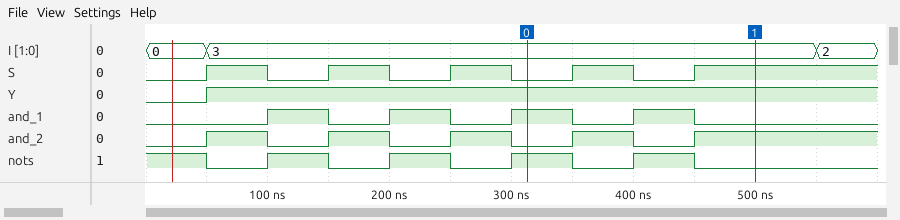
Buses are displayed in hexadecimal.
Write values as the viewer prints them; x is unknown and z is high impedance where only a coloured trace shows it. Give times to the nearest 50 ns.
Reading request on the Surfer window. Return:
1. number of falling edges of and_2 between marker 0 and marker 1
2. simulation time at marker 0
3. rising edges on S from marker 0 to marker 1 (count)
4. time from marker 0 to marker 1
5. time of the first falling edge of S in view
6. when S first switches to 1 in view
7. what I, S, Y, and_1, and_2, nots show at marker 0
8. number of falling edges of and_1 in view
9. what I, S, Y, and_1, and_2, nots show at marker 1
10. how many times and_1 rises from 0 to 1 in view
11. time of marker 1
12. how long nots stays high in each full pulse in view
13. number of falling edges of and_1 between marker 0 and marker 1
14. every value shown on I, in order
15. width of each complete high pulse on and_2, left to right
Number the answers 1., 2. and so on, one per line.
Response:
1. 1
2. 300 ns
3. 2
4. 200 ns
5. 100 ns
6. 50 ns
7. I=3, S=0, Y=1, and_1=1, and_2=0, nots=1
8. 4
9. I=3, S=1, Y=1, and_1=0, and_2=1, nots=0
10. 4
11. 500 ns
12. 50 ns, 50 ns, 50 ns, 50 ns
13. 2
14. 0, 3, 2
15. 50 ns, 50 ns, 50 ns, 50 ns
